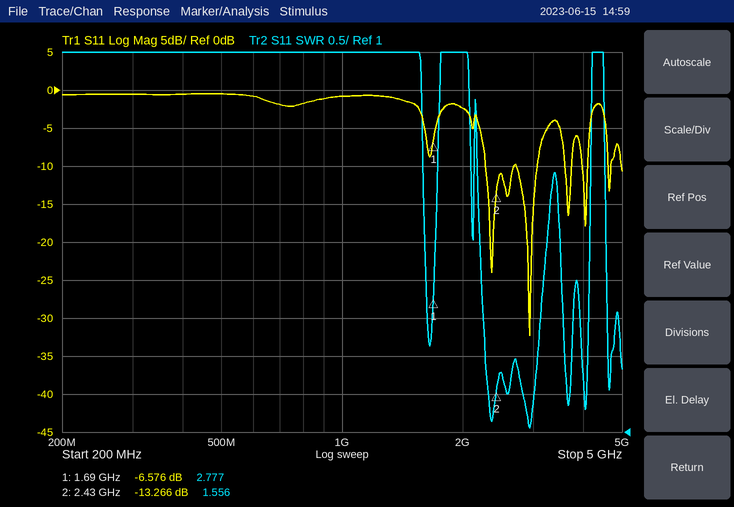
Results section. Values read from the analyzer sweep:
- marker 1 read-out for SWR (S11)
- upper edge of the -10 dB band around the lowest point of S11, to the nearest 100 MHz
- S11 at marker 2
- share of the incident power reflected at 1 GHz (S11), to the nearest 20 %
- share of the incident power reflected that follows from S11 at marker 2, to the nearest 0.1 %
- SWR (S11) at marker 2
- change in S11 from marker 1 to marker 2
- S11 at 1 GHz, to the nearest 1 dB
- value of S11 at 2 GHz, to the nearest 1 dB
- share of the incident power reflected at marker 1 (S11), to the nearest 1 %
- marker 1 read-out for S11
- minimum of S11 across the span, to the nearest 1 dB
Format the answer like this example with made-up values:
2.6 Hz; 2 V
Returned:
2.777; 3.1 GHz; -13.266 dB; 80 %; 4.7 %; 1.556; -6.690 dB; -1 dB; -2 dB; 22 %; -6.576 dB; -32 dB
